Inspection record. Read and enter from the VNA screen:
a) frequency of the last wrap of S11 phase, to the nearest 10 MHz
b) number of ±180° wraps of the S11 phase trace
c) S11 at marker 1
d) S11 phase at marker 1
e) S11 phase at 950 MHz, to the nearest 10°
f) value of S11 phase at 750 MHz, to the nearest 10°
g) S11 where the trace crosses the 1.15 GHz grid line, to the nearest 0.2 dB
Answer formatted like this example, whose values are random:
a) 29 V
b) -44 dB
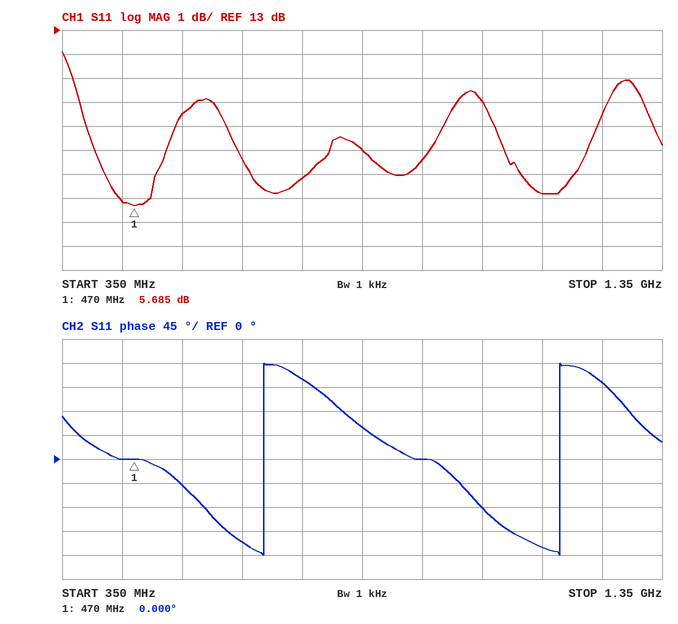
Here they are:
a) 1.18 GHz
b) 2
c) 5.685 dB
d) 0.000°
e) 0°
f) 150°
g) 6.2 dB
